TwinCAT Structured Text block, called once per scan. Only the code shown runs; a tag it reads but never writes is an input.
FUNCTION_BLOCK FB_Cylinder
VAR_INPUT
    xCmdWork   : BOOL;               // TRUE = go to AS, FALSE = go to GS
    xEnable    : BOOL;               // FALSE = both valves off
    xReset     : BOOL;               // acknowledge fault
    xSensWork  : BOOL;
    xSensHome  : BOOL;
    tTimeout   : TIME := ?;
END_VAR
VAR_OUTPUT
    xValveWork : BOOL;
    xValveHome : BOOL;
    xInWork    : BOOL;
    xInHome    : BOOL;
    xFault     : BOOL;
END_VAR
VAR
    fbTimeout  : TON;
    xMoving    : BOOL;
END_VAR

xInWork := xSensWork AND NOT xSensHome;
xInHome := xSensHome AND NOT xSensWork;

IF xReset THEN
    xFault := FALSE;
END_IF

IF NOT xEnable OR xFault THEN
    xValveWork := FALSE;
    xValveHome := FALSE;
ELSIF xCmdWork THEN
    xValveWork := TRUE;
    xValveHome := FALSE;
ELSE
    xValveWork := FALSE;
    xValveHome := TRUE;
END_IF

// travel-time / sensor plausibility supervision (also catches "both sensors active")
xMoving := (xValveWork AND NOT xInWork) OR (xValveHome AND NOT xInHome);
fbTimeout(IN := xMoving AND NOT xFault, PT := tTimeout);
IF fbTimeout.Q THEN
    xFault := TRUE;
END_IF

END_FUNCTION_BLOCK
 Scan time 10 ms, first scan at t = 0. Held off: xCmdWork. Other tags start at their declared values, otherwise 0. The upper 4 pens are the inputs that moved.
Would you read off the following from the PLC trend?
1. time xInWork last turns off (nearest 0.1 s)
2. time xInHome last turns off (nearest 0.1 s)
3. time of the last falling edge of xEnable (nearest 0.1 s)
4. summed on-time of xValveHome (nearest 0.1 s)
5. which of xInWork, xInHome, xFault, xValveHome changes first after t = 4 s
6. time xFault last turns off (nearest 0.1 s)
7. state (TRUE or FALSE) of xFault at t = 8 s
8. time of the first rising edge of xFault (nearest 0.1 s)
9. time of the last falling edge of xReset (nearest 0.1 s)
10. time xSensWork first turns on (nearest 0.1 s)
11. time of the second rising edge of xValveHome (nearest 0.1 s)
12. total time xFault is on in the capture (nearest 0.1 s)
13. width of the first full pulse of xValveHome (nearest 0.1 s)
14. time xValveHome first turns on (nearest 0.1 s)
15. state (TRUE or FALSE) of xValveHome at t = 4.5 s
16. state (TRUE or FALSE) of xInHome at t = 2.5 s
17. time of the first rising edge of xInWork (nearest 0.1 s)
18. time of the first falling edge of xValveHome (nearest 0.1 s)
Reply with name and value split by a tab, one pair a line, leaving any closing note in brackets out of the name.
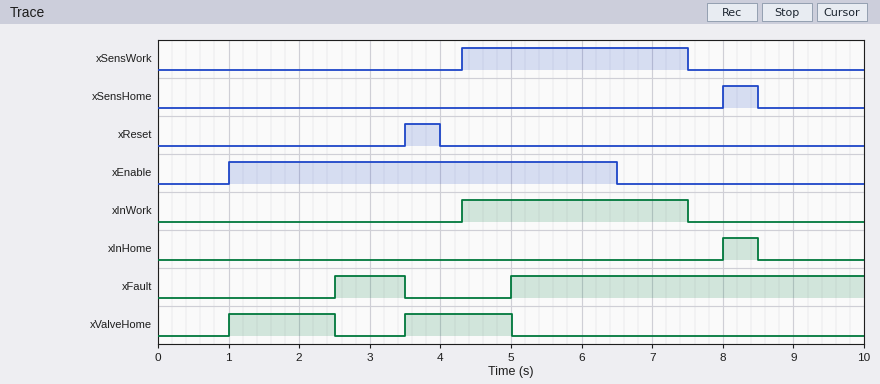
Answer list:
time xInWork last turns off	7.5 s
time xInHome last turns off	8.5 s
time of the last falling edge of xEnable	6.5 s
summed on-time of xValveHome	3.0 s
which of xInWork, xInHome, xFault, xValveHome changes first after t = 4 s	xInWork
time xFault last turns off	3.5 s
state (TRUE or FALSE) of xFault at t = 8 s	TRUE
time of the first rising edge of xFault	2.5 s
time of the last falling edge of xReset	4.0 s
time xSensWork first turns on	4.3 s
time of the second rising edge of xValveHome	3.5 s
total time xFault is on in the capture	6.0 s
width of the first full pulse of xValveHome	1.5 s
time xValveHome first turns on	1.0 s
state (TRUE or FALSE) of xValveHome at t = 4.5 s	TRUE
state (TRUE or FALSE) of xInHome at t = 2.5 s	FALSE
time of the first rising edge of xInWork	4.3 s
time of the first falling edge of xValveHome	2.5 s
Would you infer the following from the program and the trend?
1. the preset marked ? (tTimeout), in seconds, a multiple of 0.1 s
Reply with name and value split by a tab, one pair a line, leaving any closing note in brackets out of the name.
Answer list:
the preset marked ? (tTimeout), in seconds, a multiple of 0.1 s	1.5 s
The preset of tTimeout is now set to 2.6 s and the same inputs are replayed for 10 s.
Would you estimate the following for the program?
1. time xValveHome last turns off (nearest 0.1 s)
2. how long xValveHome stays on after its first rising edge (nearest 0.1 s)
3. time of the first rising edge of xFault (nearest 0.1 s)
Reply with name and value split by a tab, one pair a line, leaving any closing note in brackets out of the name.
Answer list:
time xValveHome last turns off	4.0 s
how long xValveHome stays on after its first rising edge	3.0 s
time of the first rising edge of xFault	3.6 s
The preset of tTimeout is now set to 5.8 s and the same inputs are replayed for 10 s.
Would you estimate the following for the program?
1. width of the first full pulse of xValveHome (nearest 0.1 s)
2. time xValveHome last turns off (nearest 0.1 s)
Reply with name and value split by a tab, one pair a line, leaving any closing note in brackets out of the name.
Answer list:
width of the first full pulse of xValveHome	5.5 s
time xValveHome last turns off	6.5 s
